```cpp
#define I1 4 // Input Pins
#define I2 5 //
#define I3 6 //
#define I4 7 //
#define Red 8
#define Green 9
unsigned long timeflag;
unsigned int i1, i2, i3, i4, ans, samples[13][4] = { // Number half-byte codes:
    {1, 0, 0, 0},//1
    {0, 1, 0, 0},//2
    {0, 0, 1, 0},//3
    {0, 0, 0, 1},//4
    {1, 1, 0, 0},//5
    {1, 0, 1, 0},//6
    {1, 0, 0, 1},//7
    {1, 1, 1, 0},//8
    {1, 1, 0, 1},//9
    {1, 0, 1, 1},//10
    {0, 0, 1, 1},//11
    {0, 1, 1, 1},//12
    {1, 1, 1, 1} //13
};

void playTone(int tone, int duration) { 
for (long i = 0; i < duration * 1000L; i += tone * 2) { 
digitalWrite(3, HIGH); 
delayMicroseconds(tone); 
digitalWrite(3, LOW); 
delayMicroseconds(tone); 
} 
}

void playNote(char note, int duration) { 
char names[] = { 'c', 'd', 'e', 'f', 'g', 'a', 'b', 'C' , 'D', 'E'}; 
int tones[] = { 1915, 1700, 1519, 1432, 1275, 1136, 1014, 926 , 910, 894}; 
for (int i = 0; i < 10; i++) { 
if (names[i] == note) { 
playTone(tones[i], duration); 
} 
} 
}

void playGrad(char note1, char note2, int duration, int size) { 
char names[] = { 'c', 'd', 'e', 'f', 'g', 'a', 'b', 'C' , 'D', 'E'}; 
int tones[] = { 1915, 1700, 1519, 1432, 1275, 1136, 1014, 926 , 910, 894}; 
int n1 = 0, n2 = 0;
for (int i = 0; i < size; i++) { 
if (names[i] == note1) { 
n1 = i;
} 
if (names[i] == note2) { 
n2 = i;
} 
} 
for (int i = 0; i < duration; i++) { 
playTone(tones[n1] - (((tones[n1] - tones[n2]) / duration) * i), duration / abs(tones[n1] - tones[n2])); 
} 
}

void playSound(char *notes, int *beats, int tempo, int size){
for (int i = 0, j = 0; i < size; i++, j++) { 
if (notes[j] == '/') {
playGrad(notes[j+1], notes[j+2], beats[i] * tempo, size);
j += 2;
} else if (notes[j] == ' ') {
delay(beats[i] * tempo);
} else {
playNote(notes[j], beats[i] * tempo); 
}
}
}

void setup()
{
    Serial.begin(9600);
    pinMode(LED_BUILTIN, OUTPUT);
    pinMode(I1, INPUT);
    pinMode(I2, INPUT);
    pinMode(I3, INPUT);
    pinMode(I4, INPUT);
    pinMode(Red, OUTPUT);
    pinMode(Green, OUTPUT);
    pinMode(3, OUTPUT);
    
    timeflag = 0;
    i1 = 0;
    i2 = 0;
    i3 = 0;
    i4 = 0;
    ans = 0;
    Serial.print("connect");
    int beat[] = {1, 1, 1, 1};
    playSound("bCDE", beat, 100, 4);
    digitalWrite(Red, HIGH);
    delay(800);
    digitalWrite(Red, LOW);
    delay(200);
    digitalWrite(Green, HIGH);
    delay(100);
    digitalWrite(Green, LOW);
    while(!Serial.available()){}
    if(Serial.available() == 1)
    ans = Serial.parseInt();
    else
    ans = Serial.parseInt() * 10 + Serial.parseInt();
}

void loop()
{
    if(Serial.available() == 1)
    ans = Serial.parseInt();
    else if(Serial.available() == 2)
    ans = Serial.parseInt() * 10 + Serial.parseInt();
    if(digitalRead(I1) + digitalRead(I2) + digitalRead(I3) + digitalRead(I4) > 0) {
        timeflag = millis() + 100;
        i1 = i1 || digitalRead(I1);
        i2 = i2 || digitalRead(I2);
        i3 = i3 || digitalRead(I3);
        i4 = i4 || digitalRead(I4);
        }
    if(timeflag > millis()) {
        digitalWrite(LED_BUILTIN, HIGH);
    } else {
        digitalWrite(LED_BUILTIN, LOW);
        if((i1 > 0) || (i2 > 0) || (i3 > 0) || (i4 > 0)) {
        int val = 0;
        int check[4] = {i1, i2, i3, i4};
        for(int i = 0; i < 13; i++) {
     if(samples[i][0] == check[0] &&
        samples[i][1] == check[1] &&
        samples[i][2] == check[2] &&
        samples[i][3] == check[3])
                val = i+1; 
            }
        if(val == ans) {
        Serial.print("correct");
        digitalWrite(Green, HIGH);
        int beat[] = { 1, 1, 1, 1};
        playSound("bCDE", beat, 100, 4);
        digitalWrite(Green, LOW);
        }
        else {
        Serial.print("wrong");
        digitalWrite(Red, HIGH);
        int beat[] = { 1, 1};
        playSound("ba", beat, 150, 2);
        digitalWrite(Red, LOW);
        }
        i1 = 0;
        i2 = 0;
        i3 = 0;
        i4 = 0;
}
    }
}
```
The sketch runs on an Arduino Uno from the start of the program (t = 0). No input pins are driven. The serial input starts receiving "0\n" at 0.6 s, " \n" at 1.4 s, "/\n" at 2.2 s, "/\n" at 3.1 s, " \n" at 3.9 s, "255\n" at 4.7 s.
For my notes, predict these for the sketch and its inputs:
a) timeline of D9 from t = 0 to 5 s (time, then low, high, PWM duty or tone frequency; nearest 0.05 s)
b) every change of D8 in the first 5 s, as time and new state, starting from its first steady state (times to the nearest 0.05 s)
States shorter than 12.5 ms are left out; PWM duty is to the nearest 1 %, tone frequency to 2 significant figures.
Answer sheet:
0 s low; 1.4 s high; 1.5 s low
0 s low; 0.4 s high; 1.2 s low
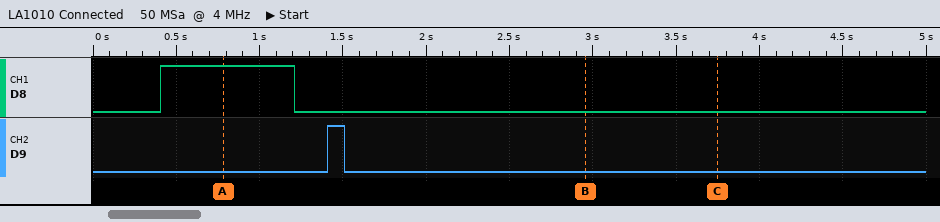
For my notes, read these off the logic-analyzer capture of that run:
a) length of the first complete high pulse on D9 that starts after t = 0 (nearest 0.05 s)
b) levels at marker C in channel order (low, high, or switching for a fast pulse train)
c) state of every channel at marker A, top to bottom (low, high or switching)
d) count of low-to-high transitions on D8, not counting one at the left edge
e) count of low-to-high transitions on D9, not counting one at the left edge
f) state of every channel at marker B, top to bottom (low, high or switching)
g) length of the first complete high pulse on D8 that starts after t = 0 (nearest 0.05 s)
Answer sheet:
0.10 s
D8 low, D9 low
D8 high, D9 low
1
1
D8 low, D9 low
0.80 s
